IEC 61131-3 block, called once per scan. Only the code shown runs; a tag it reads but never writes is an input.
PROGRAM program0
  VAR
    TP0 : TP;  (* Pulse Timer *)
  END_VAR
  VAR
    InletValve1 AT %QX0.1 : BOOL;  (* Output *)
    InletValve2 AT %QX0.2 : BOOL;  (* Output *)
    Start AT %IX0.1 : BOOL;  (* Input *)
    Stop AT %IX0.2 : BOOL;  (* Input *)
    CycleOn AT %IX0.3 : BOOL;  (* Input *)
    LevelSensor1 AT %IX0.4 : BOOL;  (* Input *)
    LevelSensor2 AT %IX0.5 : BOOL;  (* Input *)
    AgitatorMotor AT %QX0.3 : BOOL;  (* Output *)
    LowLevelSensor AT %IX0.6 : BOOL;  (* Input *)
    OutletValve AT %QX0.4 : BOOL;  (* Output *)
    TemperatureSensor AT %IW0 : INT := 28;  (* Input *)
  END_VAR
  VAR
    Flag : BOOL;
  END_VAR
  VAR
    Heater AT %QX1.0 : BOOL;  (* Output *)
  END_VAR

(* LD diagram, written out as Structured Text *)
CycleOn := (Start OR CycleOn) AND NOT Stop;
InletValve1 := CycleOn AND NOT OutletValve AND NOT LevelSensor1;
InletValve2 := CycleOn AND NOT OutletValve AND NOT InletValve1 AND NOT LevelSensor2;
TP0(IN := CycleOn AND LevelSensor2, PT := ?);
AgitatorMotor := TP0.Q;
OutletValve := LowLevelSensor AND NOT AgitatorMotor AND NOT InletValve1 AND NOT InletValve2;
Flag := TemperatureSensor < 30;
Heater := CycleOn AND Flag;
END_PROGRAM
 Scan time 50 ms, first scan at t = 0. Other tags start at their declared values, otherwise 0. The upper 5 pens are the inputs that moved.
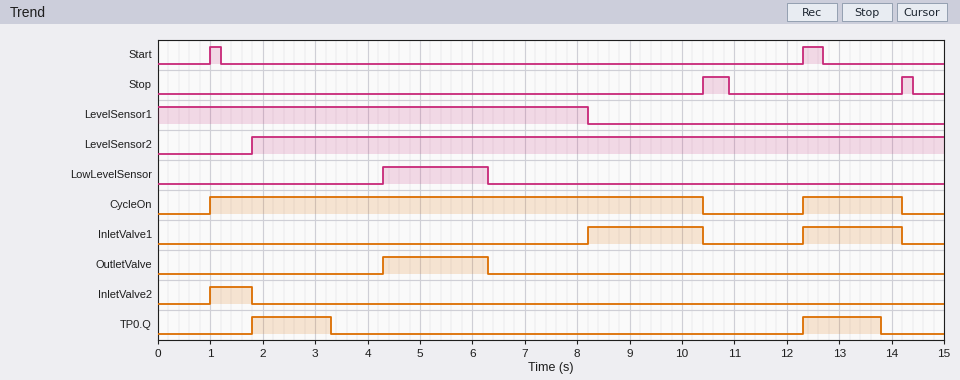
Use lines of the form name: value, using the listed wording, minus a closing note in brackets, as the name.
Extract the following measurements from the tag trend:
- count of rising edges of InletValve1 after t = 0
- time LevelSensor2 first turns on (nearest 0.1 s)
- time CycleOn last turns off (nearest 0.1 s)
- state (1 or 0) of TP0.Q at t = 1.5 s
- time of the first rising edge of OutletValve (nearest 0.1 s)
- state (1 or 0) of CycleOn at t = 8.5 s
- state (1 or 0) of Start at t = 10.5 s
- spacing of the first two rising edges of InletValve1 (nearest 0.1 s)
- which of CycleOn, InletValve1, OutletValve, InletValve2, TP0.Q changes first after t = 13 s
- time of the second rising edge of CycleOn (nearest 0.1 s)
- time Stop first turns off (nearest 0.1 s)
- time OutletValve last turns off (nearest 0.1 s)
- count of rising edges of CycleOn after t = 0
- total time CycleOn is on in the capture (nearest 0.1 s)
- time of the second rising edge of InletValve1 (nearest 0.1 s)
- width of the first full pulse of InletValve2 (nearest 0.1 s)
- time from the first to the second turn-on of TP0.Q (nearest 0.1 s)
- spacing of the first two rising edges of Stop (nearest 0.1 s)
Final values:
count of rising edges of InletValve1 after t = 0: 2
time LevelSensor2 first turns on: 1.8 s
time CycleOn last turns off: 14.2 s
state (1 or 0) of TP0.Q at t = 1.5 s: 0
time of the first rising edge of OutletValve: 4.3 s
state (1 or 0) of CycleOn at t = 8.5 s: 1
state (1 or 0) of Start at t = 10.5 s: 0
spacing of the first two rising edges of InletValve1: 4.1 s
which of CycleOn, InletValve1, OutletValve, InletValve2, TP0.Q changes first after t = 13 s: TP0.Q
time of the second rising edge of CycleOn: 12.3 s
time Stop first turns off: 10.9 s
time OutletValve last turns off: 6.3 s
count of rising edges of CycleOn after t = 0: 2
total time CycleOn is on in the capture: 11.3 s
time of the second rising edge of InletValve1: 12.3 s
width of the first full pulse of InletValve2: 0.8 s
time from the first to the second turn-on of TP0.Q: 10.5 s
spacing of the first two rising edges of Stop: 3.8 s
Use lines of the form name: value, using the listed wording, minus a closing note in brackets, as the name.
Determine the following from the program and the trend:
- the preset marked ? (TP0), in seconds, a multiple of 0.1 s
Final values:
the preset marked ? (TP0), in seconds, a multiple of 0.1 s: 1.5 s
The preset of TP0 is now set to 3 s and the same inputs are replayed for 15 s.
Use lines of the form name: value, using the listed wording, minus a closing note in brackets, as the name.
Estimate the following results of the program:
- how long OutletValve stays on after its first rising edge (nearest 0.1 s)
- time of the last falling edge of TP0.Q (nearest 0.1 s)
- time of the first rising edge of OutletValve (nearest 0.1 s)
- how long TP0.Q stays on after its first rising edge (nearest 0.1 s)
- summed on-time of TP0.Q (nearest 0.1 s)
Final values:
how long OutletValve stays on after its first rising edge: 1.5 s
time of the last falling edge of TP0.Q: 4.8 s
time of the first rising edge of OutletValve: 4.8 s
how long TP0.Q stays on after its first rising edge: 3.0 s
summed on-time of TP0.Q: 5.7 s
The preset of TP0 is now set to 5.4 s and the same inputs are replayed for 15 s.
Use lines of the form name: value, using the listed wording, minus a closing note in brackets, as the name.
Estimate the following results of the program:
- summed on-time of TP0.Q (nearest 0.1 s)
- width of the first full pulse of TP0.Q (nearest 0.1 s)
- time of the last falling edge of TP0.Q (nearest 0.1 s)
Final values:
summed on-time of TP0.Q: 8.1 s
width of the first full pulse of TP0.Q: 5.4 s
time of the last falling edge of TP0.Q: 7.2 s
